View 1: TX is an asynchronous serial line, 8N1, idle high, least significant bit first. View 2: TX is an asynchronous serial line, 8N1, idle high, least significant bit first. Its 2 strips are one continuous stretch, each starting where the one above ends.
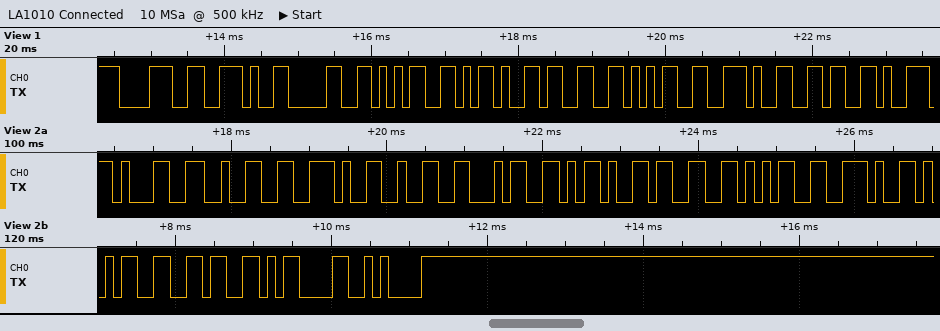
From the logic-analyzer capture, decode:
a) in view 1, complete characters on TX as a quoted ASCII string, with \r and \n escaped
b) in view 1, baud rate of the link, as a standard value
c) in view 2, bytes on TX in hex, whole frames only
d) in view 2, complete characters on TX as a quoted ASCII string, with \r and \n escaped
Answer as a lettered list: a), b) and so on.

a) "8.05-35.6"
b) 9600 baud
c) 0x31 0x32 0x2E 0x32 0x34 0x2D 0x33 0x35 0x2E 0x35 0x36 0x0D 0x0A
d) "12.24-35.56\r\n"
